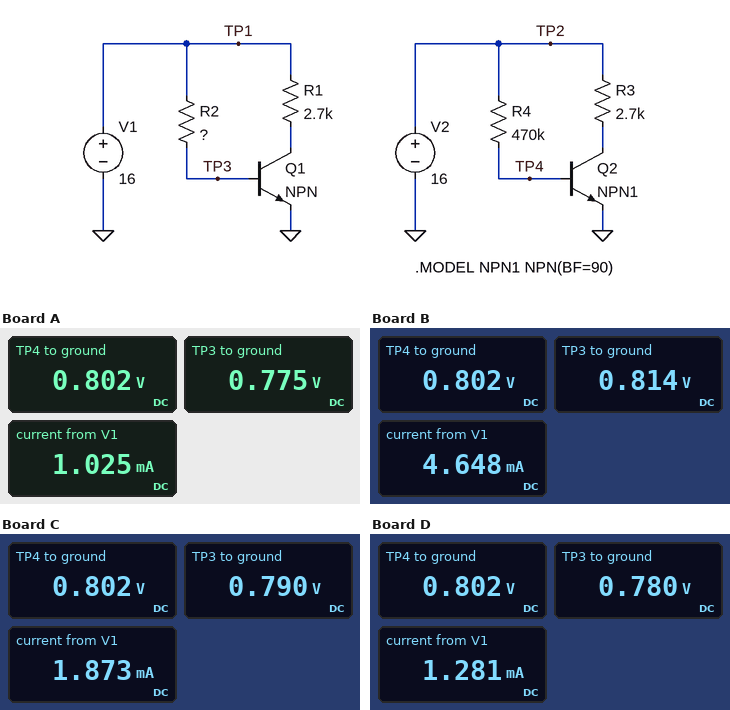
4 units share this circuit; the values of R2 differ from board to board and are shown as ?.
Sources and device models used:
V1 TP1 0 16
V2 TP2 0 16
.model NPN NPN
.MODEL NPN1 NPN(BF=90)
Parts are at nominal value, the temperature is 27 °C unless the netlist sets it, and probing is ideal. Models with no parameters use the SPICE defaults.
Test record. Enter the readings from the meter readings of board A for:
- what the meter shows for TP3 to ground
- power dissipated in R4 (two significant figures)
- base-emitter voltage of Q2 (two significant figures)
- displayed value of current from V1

0.775 V
490 µW
800 mV
1.025 mA
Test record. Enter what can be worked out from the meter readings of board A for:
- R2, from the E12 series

1.5 MΩ
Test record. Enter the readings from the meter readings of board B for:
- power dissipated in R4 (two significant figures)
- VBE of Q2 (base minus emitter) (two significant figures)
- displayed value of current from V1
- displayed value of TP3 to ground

490 µW
800 mV
4.648 mA
0.814 V
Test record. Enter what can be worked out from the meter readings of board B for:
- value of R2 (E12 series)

330 kΩ
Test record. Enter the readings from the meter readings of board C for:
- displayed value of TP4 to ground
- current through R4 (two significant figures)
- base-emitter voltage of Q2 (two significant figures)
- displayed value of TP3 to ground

0.802 V
32 µA
800 mV
0.790 V
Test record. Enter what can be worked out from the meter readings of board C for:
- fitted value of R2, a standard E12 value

820 kΩ
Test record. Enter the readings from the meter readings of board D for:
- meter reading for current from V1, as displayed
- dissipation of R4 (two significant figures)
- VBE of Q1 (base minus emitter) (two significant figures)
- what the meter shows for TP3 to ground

1.281 mA
490 µW
780 mV
0.780 V
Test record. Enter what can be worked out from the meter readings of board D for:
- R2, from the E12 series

1.2 MΩ
